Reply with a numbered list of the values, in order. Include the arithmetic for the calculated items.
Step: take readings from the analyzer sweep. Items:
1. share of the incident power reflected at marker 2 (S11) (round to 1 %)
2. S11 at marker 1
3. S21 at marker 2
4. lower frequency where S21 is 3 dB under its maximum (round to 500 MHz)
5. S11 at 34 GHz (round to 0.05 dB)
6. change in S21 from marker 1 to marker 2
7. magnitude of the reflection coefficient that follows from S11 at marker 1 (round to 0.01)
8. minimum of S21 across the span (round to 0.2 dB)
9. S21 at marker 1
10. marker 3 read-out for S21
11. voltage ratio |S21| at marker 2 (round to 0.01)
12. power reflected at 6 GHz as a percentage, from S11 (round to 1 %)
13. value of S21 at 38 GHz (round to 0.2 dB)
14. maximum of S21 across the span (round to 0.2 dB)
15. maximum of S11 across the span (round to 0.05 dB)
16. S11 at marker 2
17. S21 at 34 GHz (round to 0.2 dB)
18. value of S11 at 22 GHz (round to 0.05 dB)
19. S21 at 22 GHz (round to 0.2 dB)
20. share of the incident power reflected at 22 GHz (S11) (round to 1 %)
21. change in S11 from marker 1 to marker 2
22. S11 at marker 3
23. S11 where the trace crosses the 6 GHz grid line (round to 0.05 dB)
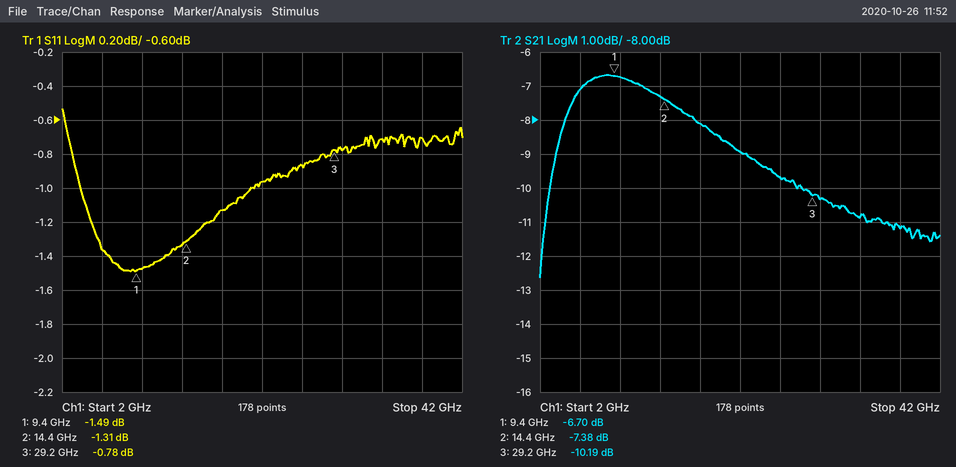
1. 10^(-1.31/10) ≈ 74 %
2. -1.49 dB
3. -7.38 dB
4. 3.0 GHz
5. -0.70 dB
6. -7.38 − (-6.7) = -0.68 dB
7. 10^(-1.49/20) ≈ 0.84
8. -12.6 dB
9. -6.70 dB
10. -10.19 dB
11. 10^(-7.38/20) ≈ 0.43
12. 10^(-1.35/10) ≈ 73 %
13. -11.2 dB
14. -6.6 dB
15. -0.55 dB
16. -1.31 dB
17. -10.8 dB
18. -0.95 dB
19. -9.0 dB
20. 10^(-0.95/10) ≈ 80 %
21. -1.31 − (-1.49) = 0.18 dB
22. -0.78 dB
23. -1.35 dB
